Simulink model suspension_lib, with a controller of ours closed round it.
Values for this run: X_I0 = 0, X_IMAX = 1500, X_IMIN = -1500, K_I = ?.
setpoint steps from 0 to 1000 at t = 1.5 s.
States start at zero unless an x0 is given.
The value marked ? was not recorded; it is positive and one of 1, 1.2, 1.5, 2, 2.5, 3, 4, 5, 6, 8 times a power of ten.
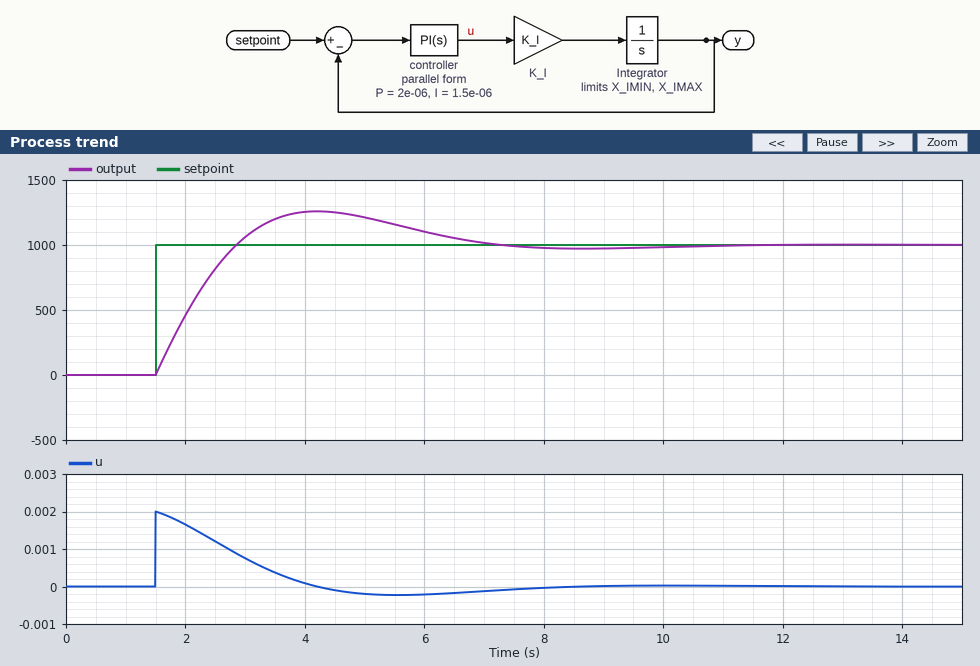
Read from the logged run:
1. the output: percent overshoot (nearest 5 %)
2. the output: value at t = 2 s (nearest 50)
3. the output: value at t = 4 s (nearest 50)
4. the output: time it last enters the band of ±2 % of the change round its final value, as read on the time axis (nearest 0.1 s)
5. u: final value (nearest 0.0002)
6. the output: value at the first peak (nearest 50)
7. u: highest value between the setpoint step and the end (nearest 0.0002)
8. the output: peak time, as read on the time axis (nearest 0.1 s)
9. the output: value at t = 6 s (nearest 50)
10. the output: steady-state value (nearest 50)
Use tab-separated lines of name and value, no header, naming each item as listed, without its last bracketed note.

the output: percent overshoot	25 %
the output: value at t = 2 s	450
the output: value at t = 4 s	1250
the output: time it last enters the band of ±2 % of the change round its final value, as read on the time axis	9.7 s
u: final value	0.0000
the output: value at the first peak	1250
u: highest value between the setpoint step and the end	0.0020
the output: peak time, as read on the time axis	4.2 s
the output: value at t = 6 s	1100
the output: steady-state value	1000
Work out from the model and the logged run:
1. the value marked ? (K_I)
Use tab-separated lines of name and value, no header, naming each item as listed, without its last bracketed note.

the value marked ?	500000
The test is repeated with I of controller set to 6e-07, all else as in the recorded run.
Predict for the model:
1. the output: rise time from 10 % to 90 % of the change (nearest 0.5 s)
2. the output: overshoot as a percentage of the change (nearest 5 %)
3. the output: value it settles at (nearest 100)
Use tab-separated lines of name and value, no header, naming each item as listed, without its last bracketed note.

the output: rise time from 10 % to 90 % of the change	1.5 s
the output: overshoot as a percentage of the change	15 %
the output: value it settles at	1000
